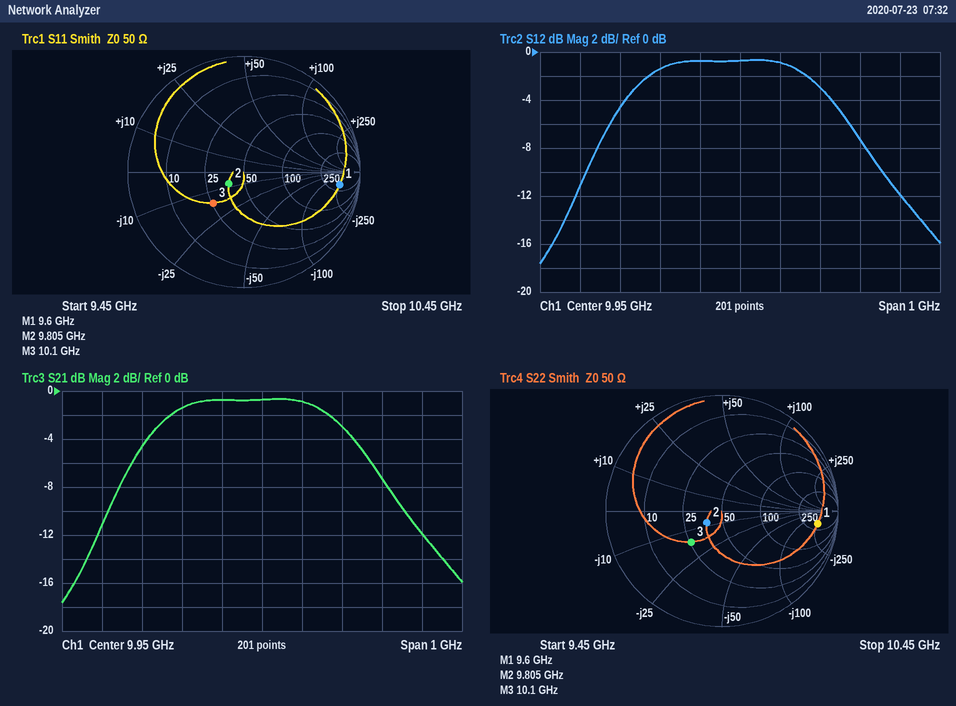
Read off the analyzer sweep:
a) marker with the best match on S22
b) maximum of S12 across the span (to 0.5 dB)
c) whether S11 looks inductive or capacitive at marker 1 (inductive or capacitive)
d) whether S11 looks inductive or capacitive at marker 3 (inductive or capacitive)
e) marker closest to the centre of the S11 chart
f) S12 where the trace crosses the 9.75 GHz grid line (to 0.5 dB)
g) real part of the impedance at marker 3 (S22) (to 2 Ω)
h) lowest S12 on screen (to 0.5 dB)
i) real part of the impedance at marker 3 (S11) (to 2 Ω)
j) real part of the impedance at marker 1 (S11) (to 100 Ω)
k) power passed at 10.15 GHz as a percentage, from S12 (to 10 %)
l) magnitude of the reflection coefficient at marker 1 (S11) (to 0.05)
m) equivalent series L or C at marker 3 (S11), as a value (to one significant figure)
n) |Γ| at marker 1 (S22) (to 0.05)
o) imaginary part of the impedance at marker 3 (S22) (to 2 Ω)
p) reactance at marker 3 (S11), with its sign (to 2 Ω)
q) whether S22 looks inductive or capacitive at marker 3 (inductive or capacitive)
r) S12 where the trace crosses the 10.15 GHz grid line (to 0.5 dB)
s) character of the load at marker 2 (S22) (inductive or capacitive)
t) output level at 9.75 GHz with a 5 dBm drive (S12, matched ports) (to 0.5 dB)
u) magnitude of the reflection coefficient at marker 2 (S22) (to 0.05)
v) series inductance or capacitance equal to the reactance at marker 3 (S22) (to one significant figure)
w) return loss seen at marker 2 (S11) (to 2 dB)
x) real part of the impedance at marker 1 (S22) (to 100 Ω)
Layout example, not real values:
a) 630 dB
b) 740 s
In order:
a) marker 2
b) -0.5 dB
c) capacitive
d) capacitive
e) marker 2
f) -1.5 dB
g) 26 Ω
h) -17.5 dB
i) 26 Ω
j) 400 Ω
k) 50 %
l) 0.85
m) 1.0 pF
n) 0.85
o) -16 Ω
p) -16 Ω
q) capacitive
r) -3.0 dB
s) capacitive
t) 3.5 dBm
u) 0.15
v) 1.0 pF
w) 16 dB
x) 400 Ω
